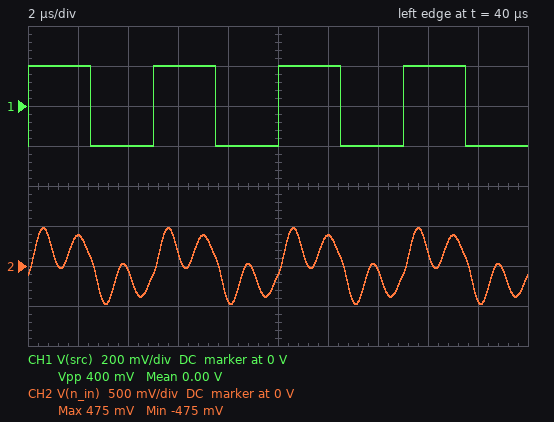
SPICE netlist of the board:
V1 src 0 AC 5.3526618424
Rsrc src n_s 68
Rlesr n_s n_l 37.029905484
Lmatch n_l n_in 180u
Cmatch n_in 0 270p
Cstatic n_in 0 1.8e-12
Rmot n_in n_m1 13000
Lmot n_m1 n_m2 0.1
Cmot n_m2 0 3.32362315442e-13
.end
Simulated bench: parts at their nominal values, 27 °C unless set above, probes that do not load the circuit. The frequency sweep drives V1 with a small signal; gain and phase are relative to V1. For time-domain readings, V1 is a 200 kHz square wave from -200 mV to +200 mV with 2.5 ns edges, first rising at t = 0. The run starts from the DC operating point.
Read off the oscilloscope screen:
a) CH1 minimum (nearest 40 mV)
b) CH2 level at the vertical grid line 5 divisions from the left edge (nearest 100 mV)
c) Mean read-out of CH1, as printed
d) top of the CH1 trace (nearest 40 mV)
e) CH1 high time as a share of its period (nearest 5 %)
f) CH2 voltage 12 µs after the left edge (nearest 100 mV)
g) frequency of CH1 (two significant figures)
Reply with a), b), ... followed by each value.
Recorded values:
a) -200 mV
b) -100 mV
c) 0.00 V
d) 200 mV
e) 50 %
f) 400 mV
g) 200 kHz
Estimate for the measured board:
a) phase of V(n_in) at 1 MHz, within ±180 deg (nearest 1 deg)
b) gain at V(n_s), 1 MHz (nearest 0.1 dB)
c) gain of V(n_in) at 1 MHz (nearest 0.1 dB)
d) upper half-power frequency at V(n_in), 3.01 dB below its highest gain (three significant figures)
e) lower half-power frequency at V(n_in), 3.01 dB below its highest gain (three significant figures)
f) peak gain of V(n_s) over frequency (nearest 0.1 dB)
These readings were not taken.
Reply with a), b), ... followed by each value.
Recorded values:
a) -169 deg
b) -0.1 dB
c) 0.5 dB
d) 760 kHz
e) 667 kHz
f) 0 dB
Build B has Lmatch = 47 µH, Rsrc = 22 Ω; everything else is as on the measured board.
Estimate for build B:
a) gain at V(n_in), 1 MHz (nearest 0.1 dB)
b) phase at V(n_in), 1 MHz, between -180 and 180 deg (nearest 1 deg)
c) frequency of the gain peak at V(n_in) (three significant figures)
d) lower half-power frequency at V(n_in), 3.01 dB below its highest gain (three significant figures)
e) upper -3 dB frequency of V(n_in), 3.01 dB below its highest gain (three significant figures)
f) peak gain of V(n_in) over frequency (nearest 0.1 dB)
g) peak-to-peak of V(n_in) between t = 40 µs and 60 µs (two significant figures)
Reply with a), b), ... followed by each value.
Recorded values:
a) 5.9 dB
b) -11 deg
c) 1.40 MHz
d) 1.30 MHz
e) 1.50 MHz
f) 17.0 dB
g) 1.2 V
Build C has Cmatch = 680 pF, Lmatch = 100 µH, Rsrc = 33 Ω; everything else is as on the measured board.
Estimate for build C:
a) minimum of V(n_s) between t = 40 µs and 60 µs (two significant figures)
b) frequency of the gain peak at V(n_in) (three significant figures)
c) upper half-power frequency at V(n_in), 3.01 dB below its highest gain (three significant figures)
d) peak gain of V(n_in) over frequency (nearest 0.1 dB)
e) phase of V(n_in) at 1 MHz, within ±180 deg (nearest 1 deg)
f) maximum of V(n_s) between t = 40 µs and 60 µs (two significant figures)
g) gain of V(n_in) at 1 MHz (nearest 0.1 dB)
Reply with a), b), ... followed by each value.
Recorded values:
a) -240 mV
b) 604 kHz
c) 658 kHz
d) 14.8 dB
e) -170 deg
f) 240 mV
g) -4.7 dB
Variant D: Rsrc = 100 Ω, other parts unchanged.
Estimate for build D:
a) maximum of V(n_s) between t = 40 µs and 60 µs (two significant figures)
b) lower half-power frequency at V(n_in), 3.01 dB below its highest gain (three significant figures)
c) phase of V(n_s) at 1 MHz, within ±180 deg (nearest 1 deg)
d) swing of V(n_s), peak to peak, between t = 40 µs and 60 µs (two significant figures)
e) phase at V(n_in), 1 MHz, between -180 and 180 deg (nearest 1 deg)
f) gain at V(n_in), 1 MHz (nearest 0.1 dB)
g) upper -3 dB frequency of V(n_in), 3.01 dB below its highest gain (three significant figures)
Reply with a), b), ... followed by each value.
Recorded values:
a) 230 mV
b) 650 kHz
c) 10 deg
d) 460 mV
e) -166 deg
f) 0.4 dB
g) 771 kHz
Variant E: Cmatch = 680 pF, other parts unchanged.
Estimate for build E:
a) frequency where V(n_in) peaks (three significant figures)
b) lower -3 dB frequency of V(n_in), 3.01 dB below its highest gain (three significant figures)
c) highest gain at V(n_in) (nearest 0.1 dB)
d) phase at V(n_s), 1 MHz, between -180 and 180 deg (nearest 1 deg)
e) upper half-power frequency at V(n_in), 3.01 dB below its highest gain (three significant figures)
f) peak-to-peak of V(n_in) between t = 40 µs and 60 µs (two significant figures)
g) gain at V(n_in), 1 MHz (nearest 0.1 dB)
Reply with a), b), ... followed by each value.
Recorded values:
a) 449 kHz
b) 400 kHz
c) 13.8 dB
d) 4 deg
e) 494 kHz
f) 810 mV
g) -11.7 dB
